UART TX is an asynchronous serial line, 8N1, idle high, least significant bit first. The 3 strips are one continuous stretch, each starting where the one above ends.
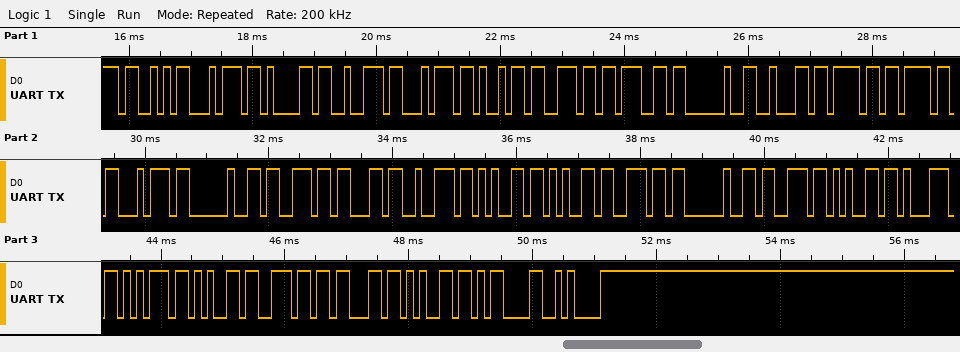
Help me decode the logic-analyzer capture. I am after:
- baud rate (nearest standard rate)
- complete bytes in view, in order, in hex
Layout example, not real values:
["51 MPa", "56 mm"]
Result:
["9600 baud", "53 74 61 72 74 69 6E 67 20 62 6F 6F 74 20 73 63 72 65 65 6E 20 73 65 71 75 65 6E 63 65 0D 0A"]
